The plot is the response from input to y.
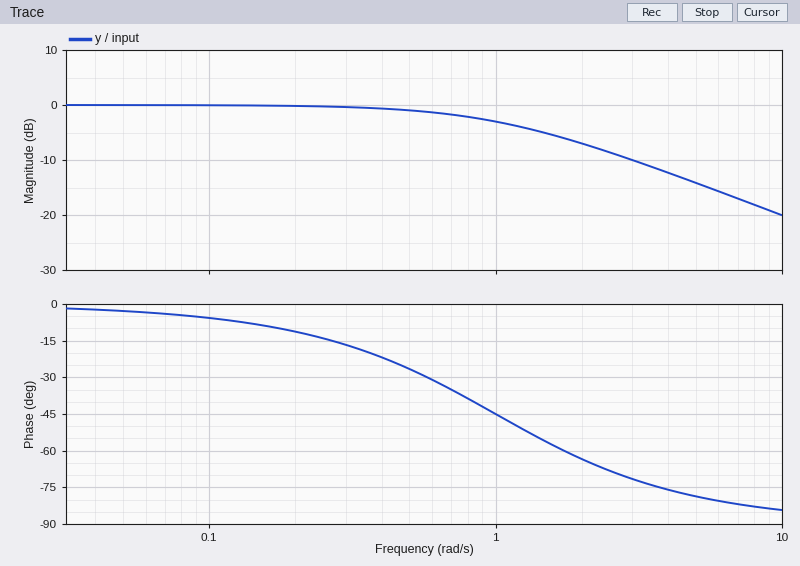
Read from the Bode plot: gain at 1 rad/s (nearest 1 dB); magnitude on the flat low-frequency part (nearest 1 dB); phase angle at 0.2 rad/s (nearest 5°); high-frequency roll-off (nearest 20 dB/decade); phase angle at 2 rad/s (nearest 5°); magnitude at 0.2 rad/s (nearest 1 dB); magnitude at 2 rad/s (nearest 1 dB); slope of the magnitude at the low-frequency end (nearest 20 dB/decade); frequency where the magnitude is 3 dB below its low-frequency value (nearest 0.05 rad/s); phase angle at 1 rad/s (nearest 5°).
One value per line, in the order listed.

-3 dB
0 dB
-10°
-20 dB/decade
-65°
0 dB
-7 dB
0 dB/decade
1.00 rad/s
-45°
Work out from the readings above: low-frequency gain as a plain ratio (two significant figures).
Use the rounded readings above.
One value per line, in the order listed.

1.0
